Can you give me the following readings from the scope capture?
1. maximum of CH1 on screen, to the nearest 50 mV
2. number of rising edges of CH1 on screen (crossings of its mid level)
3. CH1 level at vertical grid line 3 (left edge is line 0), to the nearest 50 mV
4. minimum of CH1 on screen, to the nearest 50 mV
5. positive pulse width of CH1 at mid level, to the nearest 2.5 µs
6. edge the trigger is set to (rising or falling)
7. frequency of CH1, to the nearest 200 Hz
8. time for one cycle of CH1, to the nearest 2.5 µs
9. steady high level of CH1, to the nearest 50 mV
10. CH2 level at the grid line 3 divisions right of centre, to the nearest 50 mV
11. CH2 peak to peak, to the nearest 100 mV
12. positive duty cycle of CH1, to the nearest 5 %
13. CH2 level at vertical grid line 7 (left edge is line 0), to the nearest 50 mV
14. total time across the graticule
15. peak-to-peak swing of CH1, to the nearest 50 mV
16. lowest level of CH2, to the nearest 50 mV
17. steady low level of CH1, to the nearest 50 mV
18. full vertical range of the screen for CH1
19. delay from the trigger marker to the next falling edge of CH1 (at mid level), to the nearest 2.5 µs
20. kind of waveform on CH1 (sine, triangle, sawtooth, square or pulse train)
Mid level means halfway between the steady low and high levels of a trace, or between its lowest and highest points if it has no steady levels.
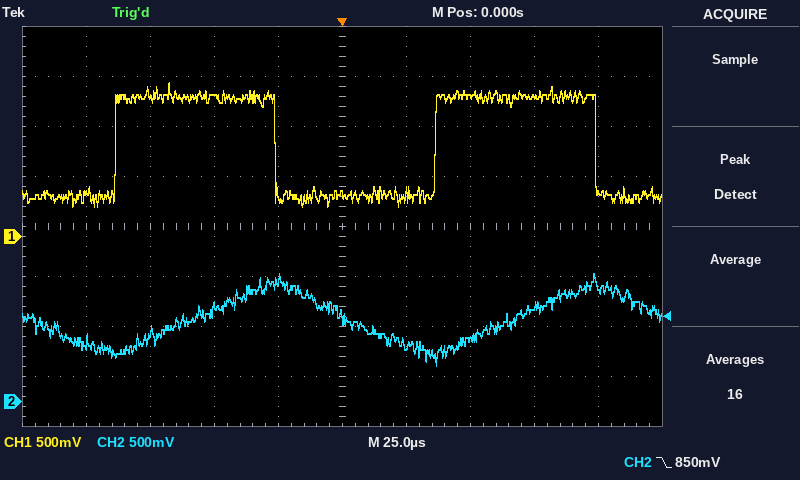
1.55 V
2
1.40 V
300 mV
62.5 µs
falling
8.0 kHz
125.0 µs
1.40 V
950 mV
900 mV
50 %
650 mV
250 µs
1.25 V
350 mV
400 mV
4 V
100.0 µs
square
